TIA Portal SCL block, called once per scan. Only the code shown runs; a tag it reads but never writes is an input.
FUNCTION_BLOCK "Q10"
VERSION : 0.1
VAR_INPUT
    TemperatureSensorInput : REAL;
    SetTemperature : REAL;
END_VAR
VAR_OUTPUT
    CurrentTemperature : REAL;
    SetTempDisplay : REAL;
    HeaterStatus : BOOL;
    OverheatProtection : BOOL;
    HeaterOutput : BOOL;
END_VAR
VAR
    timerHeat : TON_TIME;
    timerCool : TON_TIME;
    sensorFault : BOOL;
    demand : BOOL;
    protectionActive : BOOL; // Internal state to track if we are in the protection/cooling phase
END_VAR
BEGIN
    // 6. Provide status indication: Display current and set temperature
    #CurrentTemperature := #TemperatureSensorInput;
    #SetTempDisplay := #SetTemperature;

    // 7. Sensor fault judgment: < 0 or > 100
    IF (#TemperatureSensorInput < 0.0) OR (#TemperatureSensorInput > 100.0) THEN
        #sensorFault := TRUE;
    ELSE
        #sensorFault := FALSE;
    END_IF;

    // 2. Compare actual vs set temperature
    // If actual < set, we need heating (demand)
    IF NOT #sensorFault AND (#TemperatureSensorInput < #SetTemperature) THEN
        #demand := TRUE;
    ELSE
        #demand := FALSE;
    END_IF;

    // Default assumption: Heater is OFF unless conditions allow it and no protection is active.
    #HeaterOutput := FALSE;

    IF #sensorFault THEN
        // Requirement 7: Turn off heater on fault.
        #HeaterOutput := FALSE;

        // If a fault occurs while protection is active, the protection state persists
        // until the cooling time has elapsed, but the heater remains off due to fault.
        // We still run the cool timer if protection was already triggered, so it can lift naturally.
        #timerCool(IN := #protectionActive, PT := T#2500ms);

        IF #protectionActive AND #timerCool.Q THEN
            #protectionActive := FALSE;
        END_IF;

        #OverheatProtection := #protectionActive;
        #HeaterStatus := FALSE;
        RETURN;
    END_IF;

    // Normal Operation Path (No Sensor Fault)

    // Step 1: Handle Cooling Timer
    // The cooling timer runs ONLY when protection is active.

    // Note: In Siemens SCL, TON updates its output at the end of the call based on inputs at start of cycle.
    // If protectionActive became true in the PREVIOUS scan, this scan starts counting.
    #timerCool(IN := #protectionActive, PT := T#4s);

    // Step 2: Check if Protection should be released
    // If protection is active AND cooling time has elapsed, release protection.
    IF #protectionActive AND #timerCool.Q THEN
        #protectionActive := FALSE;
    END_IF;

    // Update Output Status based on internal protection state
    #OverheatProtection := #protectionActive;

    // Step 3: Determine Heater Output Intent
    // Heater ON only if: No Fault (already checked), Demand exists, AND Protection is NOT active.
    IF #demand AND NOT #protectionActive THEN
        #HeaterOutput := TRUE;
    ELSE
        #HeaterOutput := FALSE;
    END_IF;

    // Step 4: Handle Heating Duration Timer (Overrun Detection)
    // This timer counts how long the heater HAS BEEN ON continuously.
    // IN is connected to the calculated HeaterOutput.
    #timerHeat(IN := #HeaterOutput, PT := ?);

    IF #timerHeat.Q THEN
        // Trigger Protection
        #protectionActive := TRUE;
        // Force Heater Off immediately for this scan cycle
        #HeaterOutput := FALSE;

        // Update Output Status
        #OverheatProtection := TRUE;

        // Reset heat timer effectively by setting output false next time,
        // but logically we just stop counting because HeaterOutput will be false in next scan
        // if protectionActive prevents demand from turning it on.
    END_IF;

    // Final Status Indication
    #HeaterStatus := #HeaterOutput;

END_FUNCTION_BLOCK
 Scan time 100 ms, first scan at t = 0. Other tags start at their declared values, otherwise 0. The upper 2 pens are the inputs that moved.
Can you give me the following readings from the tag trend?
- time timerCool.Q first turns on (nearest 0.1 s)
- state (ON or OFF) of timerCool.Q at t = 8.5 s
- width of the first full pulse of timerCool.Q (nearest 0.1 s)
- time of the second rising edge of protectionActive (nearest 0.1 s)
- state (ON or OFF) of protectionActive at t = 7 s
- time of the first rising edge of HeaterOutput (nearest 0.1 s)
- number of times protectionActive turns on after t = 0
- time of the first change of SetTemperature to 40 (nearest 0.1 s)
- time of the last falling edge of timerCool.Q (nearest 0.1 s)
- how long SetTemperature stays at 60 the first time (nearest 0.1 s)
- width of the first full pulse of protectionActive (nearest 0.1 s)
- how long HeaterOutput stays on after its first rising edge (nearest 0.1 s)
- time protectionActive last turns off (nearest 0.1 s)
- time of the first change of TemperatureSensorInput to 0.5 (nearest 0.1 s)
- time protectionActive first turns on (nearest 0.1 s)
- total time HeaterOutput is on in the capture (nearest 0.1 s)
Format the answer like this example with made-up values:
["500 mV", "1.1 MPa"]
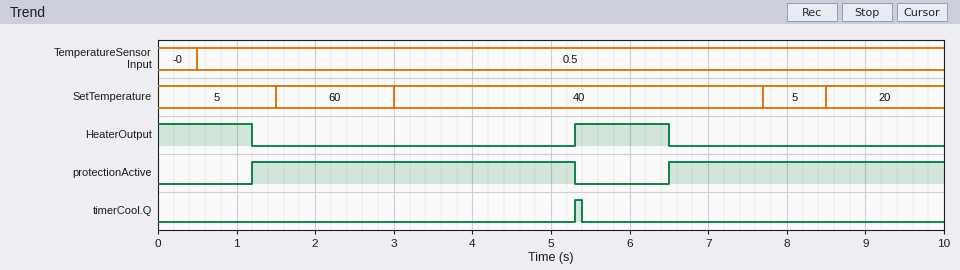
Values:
["5.3 s", "OFF", "0.1 s", "6.5 s", "ON", "5.3 s", "2", "3.0 s", "5.4 s", "1.5 s", "4.1 s", "1.2 s", "5.3 s", "0.5 s", "1.2 s", "2.4 s"]
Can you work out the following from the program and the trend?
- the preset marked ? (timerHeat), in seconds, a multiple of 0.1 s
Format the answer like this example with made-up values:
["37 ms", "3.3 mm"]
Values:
["1.2 s"]
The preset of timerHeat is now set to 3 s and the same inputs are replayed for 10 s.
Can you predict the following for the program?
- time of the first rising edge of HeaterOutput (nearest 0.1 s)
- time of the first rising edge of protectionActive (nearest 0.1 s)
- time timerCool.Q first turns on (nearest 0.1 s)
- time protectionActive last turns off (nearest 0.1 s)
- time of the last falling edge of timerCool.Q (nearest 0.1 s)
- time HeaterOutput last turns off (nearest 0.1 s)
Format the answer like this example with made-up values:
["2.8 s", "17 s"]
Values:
["7.1 s", "3.0 s", "7.1 s", "7.1 s", "7.2 s", "3.0 s"]
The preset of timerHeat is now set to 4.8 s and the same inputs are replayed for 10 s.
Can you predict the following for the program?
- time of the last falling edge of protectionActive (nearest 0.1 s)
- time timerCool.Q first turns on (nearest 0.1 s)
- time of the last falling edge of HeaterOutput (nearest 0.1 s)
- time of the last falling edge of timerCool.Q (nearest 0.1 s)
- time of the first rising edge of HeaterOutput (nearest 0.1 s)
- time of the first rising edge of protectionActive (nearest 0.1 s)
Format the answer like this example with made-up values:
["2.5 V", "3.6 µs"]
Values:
["8.9 s", "8.9 s", "4.8 s", "9.0 s", "8.9 s", "4.8 s"]
